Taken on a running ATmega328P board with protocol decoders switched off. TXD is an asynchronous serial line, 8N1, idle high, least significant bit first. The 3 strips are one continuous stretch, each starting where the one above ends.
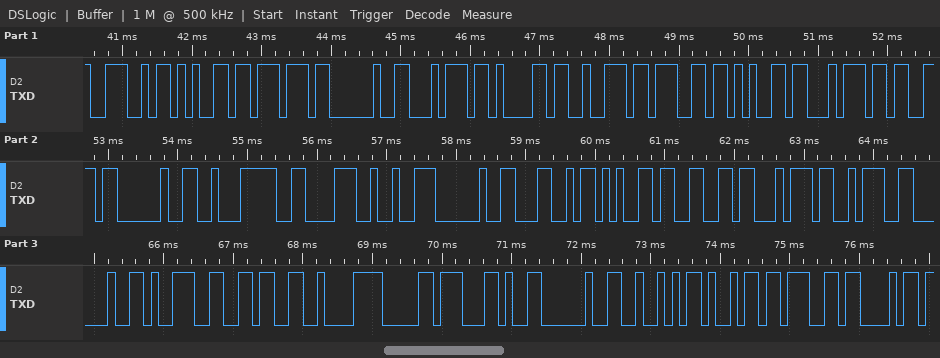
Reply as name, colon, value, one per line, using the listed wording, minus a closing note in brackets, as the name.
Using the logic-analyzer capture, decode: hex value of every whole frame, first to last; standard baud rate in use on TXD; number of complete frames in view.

hex value of every whole frame, first to last: 4E 65 77 20 74 61 72 67 65 74 73 20 E2 86 92 20 4C 65 66 74 3A 20 39 36 C2 B0 2C 20 52 69 67 68
standard baud rate in use on TXD: 9600 baud
number of complete frames in view: 32
